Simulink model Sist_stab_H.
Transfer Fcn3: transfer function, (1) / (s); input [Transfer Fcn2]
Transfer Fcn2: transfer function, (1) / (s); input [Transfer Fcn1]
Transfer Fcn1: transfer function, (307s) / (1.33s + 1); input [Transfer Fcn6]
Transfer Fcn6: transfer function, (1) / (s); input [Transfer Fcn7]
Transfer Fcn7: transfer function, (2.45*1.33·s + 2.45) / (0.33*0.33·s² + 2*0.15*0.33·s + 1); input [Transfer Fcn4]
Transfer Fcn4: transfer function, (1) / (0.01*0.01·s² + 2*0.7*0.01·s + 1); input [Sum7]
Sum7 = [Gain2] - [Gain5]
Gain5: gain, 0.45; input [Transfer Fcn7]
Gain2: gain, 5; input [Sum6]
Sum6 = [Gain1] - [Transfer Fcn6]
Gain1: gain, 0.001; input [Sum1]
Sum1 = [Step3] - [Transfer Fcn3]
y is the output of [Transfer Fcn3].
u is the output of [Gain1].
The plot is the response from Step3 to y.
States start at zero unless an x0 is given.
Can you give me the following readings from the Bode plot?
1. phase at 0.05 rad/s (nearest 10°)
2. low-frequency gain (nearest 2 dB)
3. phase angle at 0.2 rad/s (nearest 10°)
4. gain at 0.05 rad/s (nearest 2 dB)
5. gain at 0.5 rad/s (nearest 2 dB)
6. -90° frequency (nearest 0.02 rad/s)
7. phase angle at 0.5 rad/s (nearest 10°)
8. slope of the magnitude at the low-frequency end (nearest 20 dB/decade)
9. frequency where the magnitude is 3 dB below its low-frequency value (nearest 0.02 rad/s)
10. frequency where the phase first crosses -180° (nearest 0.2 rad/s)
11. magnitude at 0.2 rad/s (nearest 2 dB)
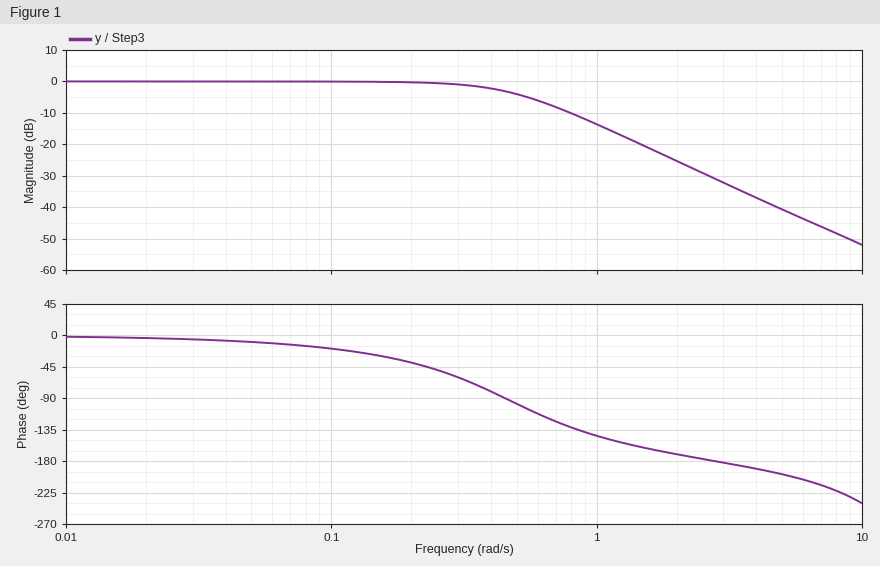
-10°
0 dB
-40°
0 dB
-4 dB
0.46 rad/s
-100°
0 dB/decade
0.44 rad/s
2.8 rad/s
0 dB
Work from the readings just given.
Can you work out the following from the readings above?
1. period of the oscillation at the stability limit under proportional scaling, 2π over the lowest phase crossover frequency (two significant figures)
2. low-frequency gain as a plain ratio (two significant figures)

2.2 s
1.0
